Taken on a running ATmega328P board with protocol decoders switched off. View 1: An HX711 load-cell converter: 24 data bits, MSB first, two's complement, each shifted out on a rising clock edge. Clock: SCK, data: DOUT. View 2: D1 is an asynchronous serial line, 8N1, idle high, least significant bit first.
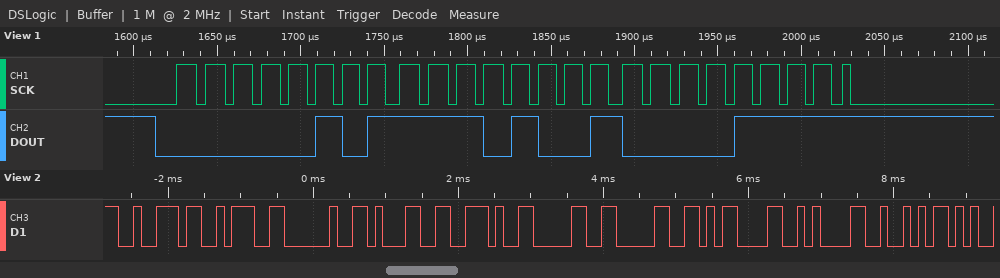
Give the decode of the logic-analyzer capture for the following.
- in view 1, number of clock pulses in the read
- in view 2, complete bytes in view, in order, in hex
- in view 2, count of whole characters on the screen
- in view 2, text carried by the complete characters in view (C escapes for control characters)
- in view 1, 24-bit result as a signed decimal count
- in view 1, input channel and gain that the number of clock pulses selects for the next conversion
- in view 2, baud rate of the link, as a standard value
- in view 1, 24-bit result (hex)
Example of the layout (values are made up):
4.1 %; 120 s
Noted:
25; 0x72 0x3A 0x20 0x31 0x2E 0x30 0x30 0x0D 0x0A 0x52; 10; "r: 1.00\r\nR"; 387343; channel A, gain 128; 9600 baud; 0x05E90F
